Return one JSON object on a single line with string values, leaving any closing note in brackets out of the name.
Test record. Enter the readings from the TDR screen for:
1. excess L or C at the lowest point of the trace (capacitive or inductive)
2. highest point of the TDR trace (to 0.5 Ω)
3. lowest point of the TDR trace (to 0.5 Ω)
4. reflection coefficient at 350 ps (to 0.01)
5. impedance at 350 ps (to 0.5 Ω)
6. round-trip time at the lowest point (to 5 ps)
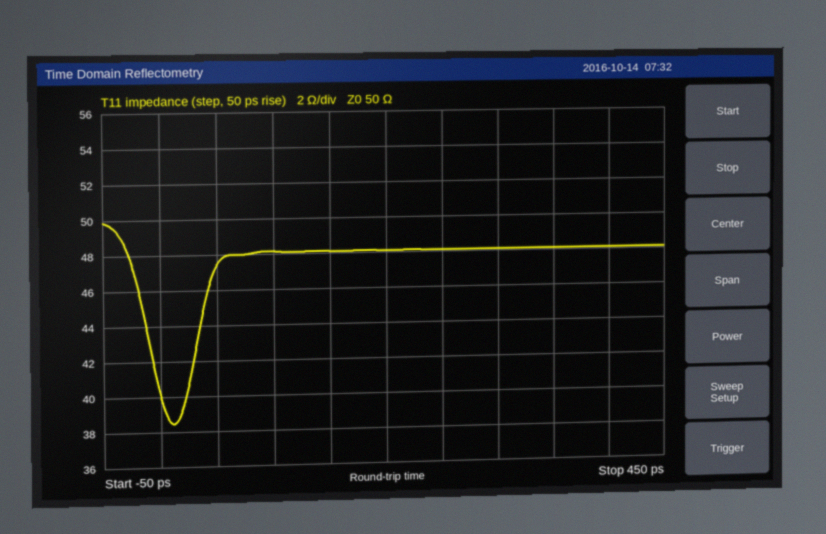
{"excess L or C at the lowest point of the trace": "capacitive", "highest point of the TDR trace": "50.0 Ω", "lowest point of the TDR trace": "38.5 Ω", "reflection coefficient at 350 ps": "-0.02", "impedance at 350 ps": "48.0 Ω", "round-trip time at the lowest point": "10 ps"}
